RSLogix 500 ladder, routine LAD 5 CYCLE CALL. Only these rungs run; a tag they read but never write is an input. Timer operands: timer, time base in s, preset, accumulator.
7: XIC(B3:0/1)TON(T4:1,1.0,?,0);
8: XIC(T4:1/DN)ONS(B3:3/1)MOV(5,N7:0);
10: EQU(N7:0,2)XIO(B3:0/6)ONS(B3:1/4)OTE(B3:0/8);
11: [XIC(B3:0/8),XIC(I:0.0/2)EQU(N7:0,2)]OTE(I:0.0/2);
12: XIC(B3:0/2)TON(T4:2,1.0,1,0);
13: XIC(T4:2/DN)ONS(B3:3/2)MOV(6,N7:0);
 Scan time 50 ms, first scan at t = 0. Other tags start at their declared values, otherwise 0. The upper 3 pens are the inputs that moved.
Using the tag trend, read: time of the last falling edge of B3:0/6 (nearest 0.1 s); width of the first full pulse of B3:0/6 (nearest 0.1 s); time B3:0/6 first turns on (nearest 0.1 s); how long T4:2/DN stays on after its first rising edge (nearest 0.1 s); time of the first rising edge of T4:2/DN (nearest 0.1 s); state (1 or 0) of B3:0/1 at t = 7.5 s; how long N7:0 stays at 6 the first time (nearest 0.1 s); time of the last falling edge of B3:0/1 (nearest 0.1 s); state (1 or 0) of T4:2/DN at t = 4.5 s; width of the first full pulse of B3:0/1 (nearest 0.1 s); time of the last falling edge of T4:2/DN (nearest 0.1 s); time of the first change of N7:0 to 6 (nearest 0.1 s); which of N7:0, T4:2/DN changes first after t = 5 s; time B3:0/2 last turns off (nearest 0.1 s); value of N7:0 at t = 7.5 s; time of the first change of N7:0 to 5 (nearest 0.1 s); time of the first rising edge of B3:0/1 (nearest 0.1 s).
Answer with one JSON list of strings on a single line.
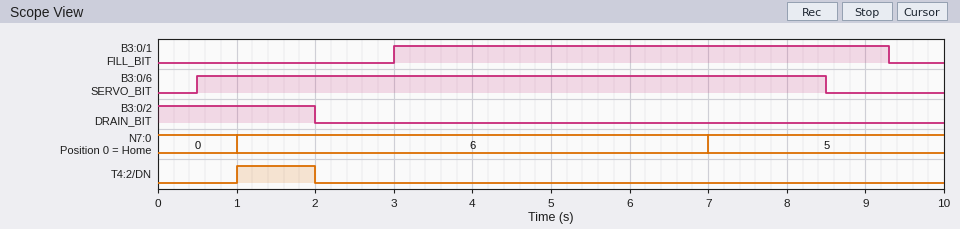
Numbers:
["8.5 s", "8.0 s", "0.5 s", "1.0 s", "1.0 s", "1", "6.0 s", "9.3 s", "0", "6.3 s", "2.0 s", "1.0 s", "N7:0", "2.0 s", "5", "7.0 s", "3.0 s"]
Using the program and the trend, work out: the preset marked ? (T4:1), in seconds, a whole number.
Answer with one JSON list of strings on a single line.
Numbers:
["4 s"]
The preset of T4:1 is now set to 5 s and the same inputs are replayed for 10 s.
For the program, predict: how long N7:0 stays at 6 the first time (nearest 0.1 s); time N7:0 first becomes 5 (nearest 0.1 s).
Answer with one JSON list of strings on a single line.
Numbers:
["7.0 s", "8.0 s"]
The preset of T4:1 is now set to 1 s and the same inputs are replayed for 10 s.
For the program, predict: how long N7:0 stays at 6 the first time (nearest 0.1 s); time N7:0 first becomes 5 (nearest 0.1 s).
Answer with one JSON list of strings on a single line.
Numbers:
["3.0 s", "4.0 s"]
